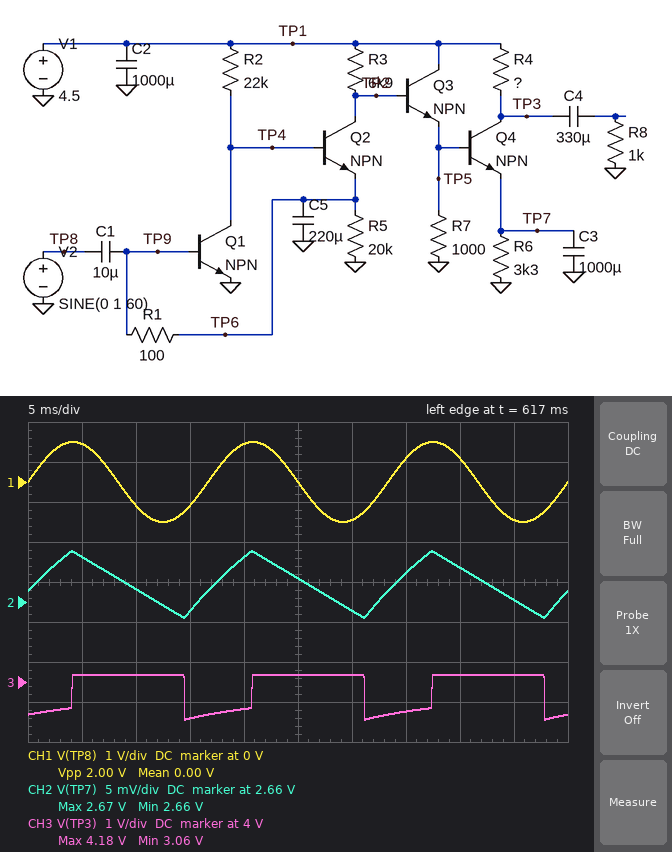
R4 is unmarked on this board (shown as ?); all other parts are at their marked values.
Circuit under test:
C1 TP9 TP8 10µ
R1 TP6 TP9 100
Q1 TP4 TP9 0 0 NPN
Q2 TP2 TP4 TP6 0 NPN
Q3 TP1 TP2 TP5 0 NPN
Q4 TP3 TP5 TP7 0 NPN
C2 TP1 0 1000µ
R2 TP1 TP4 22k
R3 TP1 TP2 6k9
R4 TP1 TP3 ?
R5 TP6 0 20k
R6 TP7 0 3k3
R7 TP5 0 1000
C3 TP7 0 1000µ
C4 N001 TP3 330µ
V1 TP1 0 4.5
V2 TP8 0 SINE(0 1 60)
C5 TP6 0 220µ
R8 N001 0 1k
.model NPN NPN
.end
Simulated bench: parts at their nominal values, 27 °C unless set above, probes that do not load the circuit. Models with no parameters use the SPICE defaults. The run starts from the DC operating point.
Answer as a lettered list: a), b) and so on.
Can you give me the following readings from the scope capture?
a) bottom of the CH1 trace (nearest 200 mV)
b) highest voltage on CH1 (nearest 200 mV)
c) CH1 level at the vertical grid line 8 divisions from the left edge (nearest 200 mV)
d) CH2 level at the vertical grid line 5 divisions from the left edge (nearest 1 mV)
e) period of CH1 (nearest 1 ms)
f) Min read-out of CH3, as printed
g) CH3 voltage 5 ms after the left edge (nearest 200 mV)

a) -1.0 V
b) 1.0 V
c) 600 mV
d) 2.663 V
e) 17 ms
f) 3.06 V
g) 4.2 V
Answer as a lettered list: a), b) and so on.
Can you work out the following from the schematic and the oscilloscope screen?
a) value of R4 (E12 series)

a) 820 Ω
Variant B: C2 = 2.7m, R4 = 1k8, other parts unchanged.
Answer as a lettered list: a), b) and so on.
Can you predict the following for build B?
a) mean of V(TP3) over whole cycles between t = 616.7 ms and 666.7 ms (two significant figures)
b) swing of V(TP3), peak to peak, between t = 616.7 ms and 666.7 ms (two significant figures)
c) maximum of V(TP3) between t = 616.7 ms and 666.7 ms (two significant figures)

a) 3.3 V
b) 1.1 V
c) 3.7 V
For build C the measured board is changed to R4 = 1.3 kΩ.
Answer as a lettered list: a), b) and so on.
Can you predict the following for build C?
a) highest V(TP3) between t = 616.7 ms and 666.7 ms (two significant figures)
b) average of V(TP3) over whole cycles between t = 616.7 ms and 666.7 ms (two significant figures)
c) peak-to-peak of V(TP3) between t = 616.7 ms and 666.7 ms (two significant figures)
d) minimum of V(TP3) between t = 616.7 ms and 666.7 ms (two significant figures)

a) 3.9 V
b) 3.5 V
c) 1.2 V
d) 2.7 V
